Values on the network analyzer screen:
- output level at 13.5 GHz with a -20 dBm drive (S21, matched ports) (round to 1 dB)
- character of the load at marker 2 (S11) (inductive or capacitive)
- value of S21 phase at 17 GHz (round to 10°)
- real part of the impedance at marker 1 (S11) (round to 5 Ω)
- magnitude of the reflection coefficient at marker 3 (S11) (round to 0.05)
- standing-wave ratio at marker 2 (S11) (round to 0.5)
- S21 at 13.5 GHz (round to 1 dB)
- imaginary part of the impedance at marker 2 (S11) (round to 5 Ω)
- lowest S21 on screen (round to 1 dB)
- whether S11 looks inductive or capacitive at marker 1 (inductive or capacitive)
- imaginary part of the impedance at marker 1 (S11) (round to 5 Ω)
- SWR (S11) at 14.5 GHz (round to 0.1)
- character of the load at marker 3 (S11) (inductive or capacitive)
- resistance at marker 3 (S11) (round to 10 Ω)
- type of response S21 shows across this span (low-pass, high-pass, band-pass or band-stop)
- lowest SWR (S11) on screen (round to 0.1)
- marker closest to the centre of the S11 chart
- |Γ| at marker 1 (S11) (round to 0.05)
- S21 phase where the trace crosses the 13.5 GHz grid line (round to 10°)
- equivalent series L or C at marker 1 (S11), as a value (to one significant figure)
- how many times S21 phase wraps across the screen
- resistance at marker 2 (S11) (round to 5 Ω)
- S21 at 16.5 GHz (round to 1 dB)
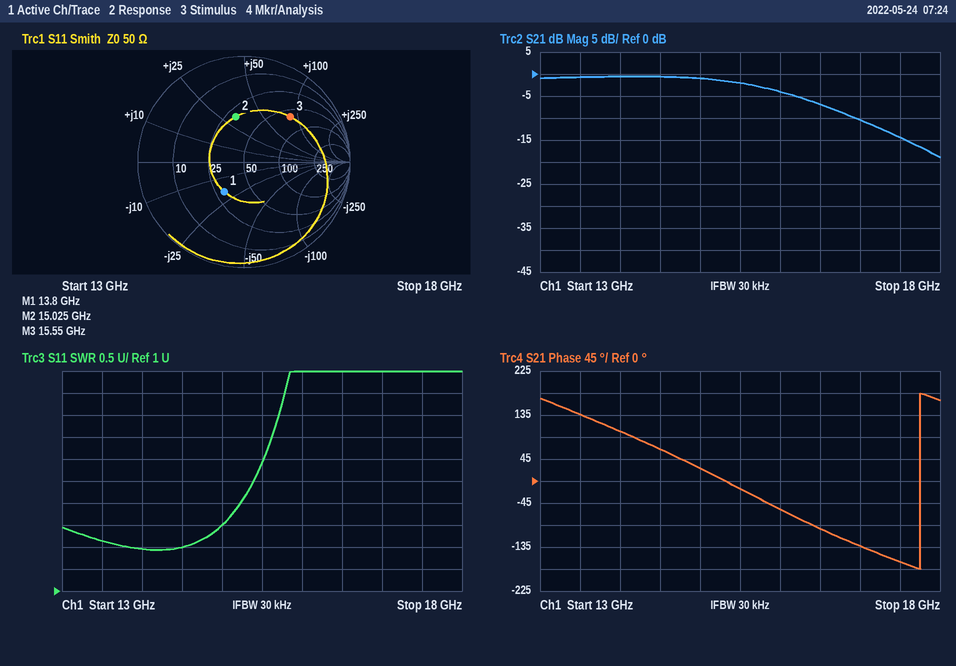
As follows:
-21 dBm
inductive
-130°
30 Ω
0.60
2.5
-1 dB
+30 Ω
-19 dB
capacitive
-20 Ω
2.0
inductive
60 Ω
low-pass
1.9
marker 1
0.35
140°
600 fF
1
30 Ω
-7 dB
